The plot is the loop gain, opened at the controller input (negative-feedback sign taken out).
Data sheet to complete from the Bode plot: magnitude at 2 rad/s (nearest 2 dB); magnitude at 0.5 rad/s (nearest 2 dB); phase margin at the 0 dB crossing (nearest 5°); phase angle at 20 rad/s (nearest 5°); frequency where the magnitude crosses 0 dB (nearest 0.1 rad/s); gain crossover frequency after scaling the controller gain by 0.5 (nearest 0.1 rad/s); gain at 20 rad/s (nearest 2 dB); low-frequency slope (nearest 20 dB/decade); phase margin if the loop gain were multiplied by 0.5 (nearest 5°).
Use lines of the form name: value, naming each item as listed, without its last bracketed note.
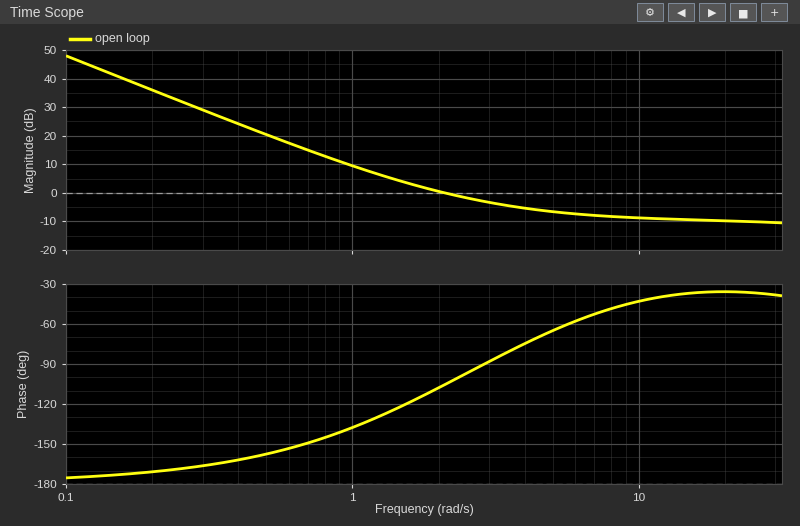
magnitude at 2 rad/s: 0 dB
magnitude at 0.5 rad/s: 20 dB
phase margin at the 0 dB crossing: 75°
phase angle at 20 rad/s: -35°
frequency where the magnitude crosses 0 dB: 2.1 rad/s
gain crossover frequency after scaling the controller gain by 0.5: 1.3 rad/s
gain at 20 rad/s: -10 dB
low-frequency slope: -40 dB/decade
phase margin if the loop gain were multiplied by 0.5: 50°
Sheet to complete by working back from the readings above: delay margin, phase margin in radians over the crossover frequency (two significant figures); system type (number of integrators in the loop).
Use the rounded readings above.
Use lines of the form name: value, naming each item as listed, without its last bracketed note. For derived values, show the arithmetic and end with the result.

delay margin, phase margin in radians over the crossover frequency: 75 × π / 180 / 2.1 = 0.62 s
system type: 2
